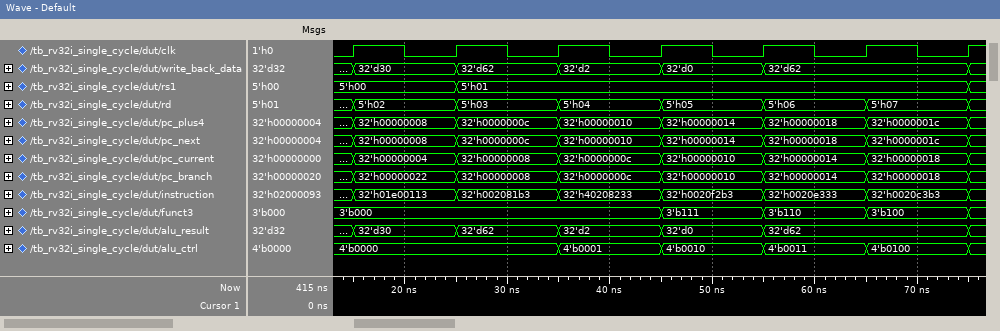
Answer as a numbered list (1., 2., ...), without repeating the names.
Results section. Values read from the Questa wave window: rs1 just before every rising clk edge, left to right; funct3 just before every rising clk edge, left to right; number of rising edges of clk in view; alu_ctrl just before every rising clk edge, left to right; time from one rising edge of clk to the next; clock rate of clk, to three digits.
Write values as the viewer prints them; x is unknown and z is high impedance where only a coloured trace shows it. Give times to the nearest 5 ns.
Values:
1. 5'h00, 5'h00, 5'h01, 5'h01, 5'h01, 5'h01, 5'h01
2. 3'b000, 3'b000, 3'b000, 3'b000, 3'b111, 3'b110, 3'b100
3. 7
4. 4'b0000, 4'b0000, 4'b0000, 4'b0001, 4'b0010, 4'b0011, 4'b0100
5. 10 ns
6. 100 MHz
